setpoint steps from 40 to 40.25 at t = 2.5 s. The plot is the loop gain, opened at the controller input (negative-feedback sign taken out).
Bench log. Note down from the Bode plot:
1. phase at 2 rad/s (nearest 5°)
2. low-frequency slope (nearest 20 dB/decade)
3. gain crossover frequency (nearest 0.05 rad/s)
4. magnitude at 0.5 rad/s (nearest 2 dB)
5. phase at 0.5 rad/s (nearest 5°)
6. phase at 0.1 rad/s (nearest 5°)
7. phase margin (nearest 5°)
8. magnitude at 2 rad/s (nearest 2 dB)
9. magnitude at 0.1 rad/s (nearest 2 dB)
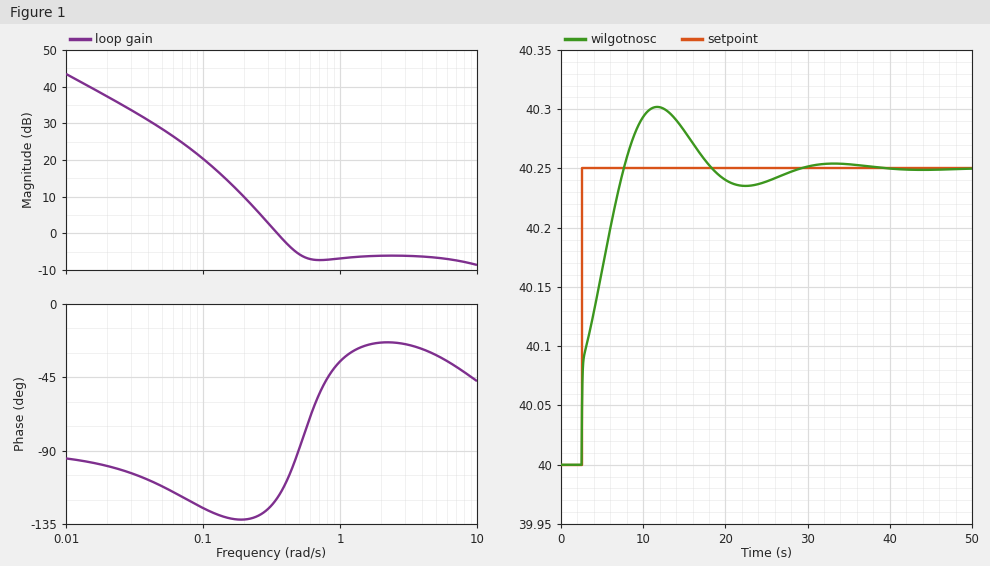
-25°
-20 dB/decade
0.35 rad/s
-6 dB
-90°
-125°
60°
-6 dB
20 dB
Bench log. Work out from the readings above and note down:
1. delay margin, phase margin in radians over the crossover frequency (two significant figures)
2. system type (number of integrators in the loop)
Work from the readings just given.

3.0 s
1
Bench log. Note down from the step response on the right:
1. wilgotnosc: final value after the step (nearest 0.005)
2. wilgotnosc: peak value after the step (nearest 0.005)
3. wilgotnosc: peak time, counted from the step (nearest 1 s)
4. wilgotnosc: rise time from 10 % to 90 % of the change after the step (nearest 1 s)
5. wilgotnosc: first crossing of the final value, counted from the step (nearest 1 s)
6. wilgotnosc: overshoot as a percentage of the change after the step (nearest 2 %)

40.250
40.300
9 s
4 s
5 s
20 %
